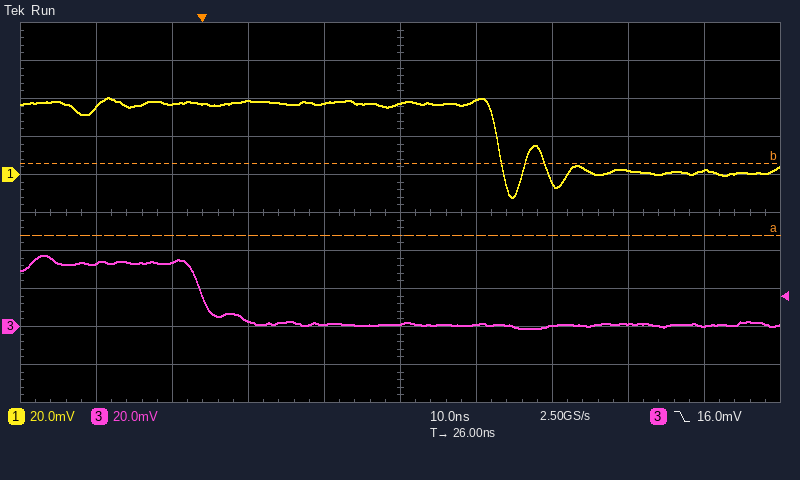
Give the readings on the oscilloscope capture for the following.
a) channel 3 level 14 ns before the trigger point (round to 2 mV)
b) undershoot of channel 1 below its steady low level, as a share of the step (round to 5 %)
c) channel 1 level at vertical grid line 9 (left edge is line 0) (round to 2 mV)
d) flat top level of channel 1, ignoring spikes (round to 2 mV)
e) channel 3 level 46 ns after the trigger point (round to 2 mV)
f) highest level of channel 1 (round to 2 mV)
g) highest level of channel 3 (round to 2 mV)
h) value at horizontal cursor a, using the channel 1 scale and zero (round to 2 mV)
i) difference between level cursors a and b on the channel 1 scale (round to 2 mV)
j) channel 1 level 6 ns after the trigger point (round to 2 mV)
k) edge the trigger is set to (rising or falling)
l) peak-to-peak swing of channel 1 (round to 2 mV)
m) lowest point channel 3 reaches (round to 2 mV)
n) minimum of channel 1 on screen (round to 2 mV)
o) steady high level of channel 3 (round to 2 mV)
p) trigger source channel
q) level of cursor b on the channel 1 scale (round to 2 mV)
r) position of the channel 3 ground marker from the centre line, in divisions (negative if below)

34 mV
35 %
2 mV
38 mV
0 mV
40 mV
38 mV
-32 mV
38 mV
38 mV
falling
52 mV
-2 mV
-12 mV
34 mV
channel 3
6 mV
-3.0 div
